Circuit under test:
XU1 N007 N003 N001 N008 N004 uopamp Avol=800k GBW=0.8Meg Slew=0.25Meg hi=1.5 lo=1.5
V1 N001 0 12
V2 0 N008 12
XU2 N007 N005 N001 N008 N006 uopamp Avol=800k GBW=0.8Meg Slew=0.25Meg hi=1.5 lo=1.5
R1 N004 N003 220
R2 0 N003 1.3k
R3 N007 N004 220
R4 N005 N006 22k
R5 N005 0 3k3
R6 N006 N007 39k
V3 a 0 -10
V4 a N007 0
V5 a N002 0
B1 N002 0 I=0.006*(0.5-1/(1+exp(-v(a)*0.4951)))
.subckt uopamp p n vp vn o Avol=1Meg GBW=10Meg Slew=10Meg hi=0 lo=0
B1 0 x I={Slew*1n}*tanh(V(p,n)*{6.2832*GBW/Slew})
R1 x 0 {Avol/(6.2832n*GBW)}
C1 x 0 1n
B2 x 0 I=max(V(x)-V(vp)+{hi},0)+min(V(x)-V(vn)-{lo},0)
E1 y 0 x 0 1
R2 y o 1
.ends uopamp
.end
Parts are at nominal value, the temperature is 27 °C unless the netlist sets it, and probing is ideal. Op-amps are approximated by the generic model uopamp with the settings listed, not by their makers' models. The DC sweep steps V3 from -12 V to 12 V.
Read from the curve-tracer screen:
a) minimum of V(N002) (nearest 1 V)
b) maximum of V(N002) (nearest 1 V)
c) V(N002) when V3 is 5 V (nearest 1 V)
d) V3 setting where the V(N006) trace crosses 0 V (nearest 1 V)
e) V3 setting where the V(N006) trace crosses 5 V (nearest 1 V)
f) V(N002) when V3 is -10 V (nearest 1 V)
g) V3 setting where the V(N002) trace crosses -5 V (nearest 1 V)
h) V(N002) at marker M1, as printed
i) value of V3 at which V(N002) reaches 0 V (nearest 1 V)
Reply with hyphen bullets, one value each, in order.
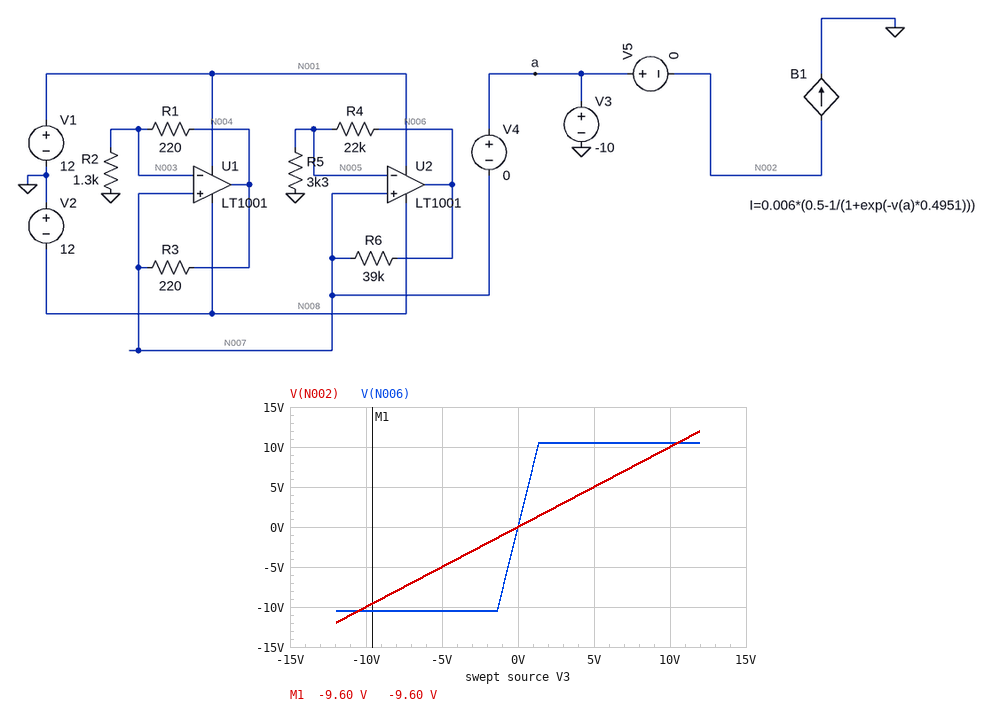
- -12 V
- 12 V
- 5 V
- 0 V
- 1 V
- -10 V
- -5 V
- -9.60 V
- 0 V
